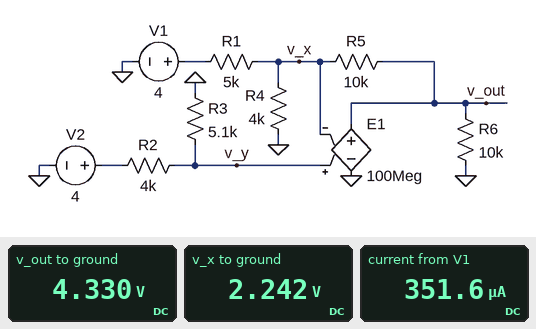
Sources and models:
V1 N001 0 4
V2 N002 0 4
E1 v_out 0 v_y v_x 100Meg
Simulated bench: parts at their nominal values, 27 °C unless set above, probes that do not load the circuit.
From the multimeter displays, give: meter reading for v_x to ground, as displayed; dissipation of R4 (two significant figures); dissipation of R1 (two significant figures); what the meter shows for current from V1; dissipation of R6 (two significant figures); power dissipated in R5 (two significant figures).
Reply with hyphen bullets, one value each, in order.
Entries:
- 2.242 V
- 1.3 mW
- 620 µW
- 351.6 µA
- 1.9 mW
- 440 µW
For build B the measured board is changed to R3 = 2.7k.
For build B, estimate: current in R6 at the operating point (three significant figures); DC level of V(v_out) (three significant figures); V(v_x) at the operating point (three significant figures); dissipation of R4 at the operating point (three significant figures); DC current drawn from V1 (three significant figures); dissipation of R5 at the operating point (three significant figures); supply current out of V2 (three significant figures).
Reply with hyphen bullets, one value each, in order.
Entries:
- 86.6 µA
- 866 mV
- 1.61 V
- 650 µW
- 478 µA
- 55.7 µW
- 597 µA
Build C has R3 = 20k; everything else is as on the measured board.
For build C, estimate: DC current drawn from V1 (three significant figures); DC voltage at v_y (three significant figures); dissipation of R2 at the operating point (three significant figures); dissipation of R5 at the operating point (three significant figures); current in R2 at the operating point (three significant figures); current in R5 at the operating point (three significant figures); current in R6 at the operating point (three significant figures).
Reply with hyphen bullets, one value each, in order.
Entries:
- 133 µA
- 3.33 V
- 111 µW
- 4.90 mW
- 167 µA
- 700 µA
- 1.03 mA
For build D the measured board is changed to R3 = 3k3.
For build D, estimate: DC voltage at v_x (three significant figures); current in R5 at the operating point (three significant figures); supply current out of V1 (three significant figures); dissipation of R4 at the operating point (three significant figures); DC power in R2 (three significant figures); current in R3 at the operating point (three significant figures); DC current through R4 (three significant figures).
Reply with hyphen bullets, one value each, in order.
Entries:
- 1.81 V
- 13.7 µA
- 438 µA
- 817 µW
- 1.20 mW
- 548 µA
- 452 µA
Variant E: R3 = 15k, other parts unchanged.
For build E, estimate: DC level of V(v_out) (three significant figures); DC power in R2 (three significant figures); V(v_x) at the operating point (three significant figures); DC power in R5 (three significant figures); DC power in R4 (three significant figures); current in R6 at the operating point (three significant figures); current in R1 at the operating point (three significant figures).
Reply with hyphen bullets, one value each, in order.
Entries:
- 9.37 V
- 177 µW
- 3.16 V
- 3.86 mW
- 2.49 mW
- 937 µA
- 168 µA
